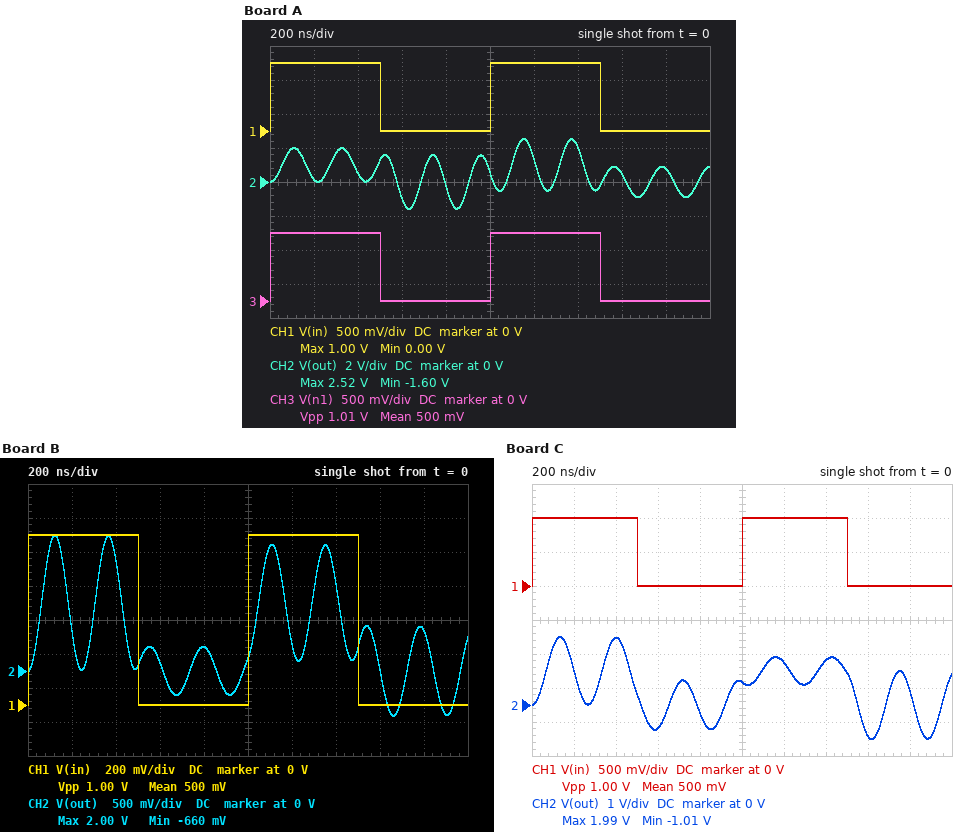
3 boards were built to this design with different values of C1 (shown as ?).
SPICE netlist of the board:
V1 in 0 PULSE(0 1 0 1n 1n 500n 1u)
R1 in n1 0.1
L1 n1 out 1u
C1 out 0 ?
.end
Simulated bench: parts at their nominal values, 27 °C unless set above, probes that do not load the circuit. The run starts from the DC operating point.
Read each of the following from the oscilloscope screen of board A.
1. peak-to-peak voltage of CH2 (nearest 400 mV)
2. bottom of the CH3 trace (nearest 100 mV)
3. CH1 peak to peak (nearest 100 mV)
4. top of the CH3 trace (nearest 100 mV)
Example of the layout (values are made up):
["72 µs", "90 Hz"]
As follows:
["4.0 V", "0 V", "1.0 V", "1.0 V"]
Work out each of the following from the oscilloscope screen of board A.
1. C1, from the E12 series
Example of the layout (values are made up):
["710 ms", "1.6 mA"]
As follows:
["1.2 nF"]
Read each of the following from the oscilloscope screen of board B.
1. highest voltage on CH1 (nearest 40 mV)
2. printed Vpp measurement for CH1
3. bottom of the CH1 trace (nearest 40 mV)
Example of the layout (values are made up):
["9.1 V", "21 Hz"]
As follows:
["1.00 V", "1.00 V", "0 V"]
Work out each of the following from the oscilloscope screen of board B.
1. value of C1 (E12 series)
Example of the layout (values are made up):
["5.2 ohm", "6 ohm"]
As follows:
["1.5 nF"]
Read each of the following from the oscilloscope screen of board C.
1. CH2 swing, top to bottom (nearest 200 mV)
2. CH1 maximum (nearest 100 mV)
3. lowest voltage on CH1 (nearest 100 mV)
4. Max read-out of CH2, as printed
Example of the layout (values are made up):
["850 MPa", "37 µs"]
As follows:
["3.0 V", "1.0 V", "0 V", "1.99 V"]
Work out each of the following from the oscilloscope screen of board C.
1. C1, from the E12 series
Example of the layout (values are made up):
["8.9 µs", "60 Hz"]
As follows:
["1.8 nF"]
